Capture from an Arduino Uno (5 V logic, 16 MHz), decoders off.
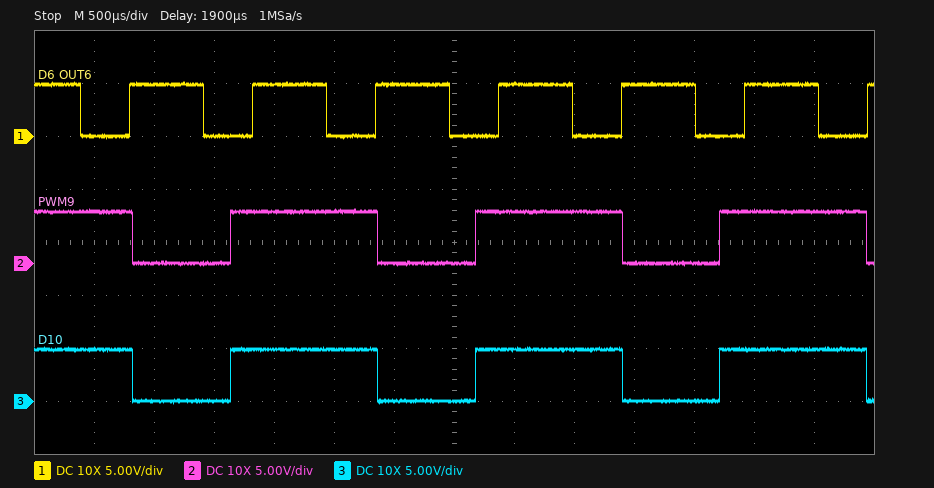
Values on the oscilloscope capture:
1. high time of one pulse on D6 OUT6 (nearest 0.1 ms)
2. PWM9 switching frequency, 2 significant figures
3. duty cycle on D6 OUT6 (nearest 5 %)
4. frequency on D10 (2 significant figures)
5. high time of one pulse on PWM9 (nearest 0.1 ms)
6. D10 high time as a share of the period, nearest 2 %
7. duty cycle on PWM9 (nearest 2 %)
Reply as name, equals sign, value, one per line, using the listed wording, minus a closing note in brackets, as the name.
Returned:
high time of one pulse on D6 OUT6 = 0.6 ms
PWM9 switching frequency, 2 significant figures = 490 Hz
duty cycle on D6 OUT6 = 60 %
frequency on D10 = 490 Hz
high time of one pulse on PWM9 = 1.2 ms
D10 high time as a share of the period, nearest 2 % = 60 %
duty cycle on PWM9 = 60 %
